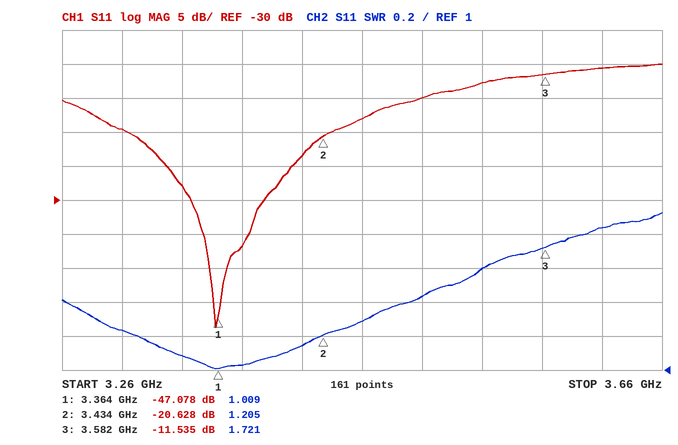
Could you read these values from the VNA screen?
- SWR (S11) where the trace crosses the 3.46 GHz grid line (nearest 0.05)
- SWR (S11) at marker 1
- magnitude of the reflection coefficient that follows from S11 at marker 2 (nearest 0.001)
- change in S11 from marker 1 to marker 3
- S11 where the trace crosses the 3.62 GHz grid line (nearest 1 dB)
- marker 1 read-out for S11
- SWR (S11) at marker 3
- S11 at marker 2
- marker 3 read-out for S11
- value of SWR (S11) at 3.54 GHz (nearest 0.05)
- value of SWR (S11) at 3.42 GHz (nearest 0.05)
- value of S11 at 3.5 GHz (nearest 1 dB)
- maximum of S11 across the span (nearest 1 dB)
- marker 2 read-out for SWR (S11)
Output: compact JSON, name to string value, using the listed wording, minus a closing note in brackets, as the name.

{"SWR (S11) where the trace crosses the 3.46 GHz grid line": "1.30", "SWR (S11) at marker 1": "1.009", "magnitude of the reflection coefficient that follows from S11 at marker 2": "0.093", "change in S11 from marker 1 to marker 3": "35.543 dB", "S11 where the trace crosses the 3.62 GHz grid line": "-11 dB", "marker 1 read-out for S11": "-47.078 dB", "SWR (S11) at marker 3": "1.721", "S11 at marker 2": "-20.628 dB", "marker 3 read-out for S11": "-11.535 dB", "value of SWR (S11) at 3.54 GHz": "1.60", "value of SWR (S11) at 3.42 GHz": "1.15", "value of S11 at 3.5 GHz": "-15 dB", "maximum of S11 across the span": "-10 dB", "marker 2 read-out for SWR": "1.205"}
